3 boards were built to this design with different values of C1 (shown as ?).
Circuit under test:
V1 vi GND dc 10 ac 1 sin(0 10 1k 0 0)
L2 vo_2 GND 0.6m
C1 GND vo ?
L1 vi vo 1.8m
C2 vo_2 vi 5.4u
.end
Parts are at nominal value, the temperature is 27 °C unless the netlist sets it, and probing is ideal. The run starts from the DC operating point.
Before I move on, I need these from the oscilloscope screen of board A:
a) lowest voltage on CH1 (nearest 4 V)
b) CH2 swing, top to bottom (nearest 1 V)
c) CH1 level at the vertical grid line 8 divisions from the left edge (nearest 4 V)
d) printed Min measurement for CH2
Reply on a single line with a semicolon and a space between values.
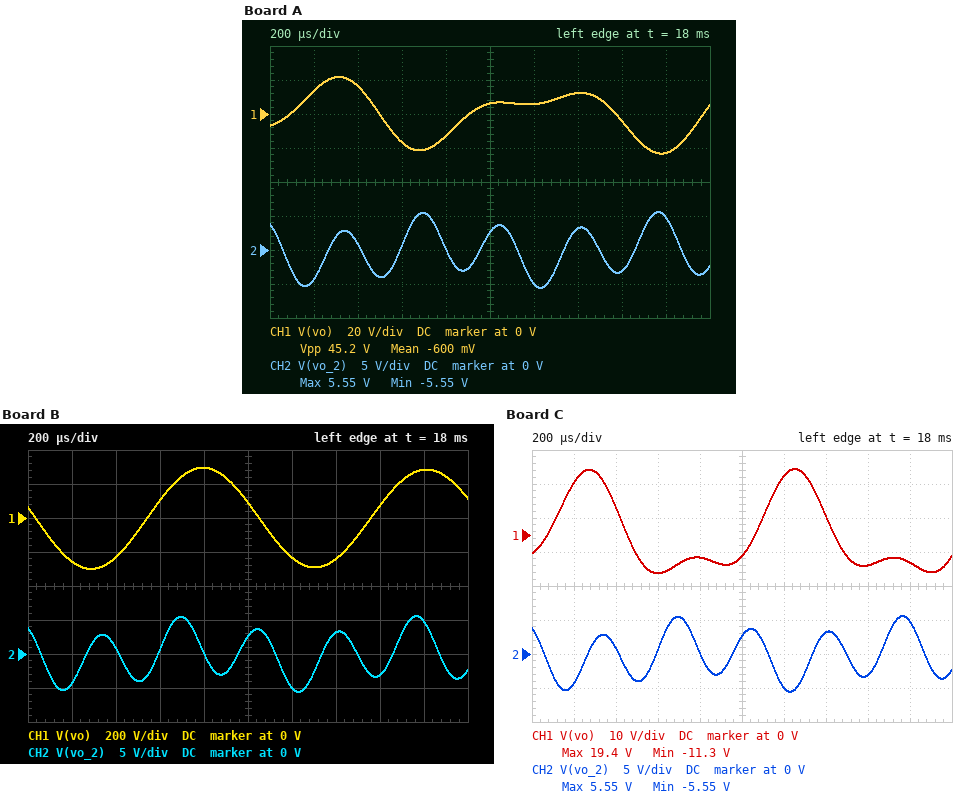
-24 V; 11 V; -4 V; -5.55 V
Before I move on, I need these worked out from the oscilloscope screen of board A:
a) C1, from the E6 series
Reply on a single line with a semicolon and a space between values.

4.7 µF
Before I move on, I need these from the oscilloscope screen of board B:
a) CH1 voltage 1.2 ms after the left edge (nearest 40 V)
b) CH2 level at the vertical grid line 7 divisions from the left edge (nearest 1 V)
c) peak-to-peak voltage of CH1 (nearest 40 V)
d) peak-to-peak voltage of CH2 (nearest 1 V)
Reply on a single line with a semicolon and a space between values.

-240 V; 3 V; 600 V; 11 V
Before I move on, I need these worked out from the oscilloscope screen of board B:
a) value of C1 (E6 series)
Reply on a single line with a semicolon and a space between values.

15 µF
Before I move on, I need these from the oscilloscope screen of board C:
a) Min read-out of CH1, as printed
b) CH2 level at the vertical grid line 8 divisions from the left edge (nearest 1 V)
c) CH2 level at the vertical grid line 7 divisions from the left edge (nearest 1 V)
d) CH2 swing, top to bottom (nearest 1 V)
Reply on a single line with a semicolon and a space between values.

-11.3 V; -3 V; 3 V; 11 V
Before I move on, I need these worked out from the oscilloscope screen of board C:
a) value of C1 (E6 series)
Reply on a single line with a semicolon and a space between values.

3.3 µF
